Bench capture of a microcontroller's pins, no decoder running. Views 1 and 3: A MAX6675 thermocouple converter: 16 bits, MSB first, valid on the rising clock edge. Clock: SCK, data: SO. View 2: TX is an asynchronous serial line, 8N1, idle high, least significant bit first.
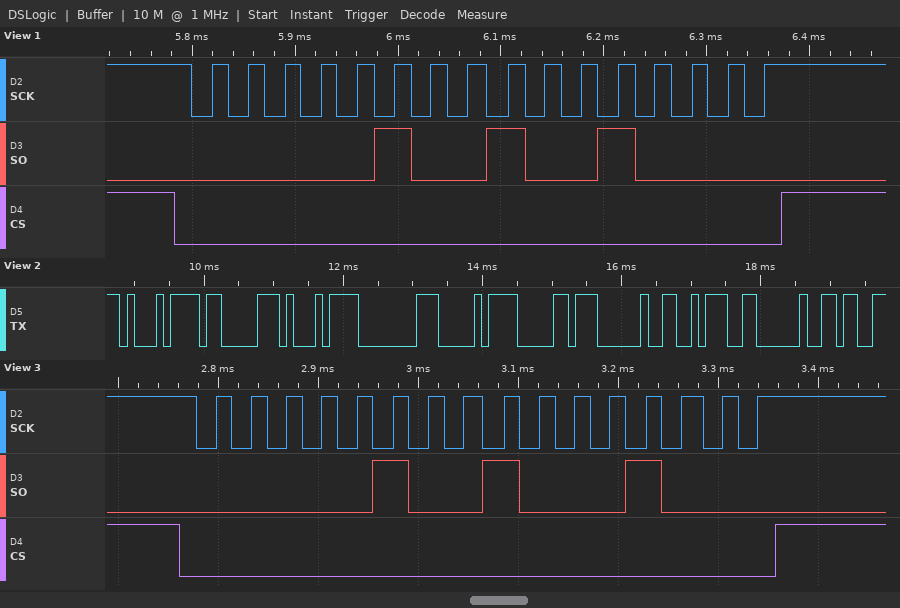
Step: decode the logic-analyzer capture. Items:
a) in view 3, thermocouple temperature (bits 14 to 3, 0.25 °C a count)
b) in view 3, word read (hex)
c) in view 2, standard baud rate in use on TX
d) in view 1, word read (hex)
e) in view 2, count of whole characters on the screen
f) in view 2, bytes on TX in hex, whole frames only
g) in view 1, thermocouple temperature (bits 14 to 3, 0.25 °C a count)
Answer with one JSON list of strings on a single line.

["36.25 °C", "0x0488", "9600 baud", "0x0490", "9", "0xD1 0x83 0xD1 0x80 0xD0 0xB0 0x20 0x3A 0x20", "36.50 °C"]
